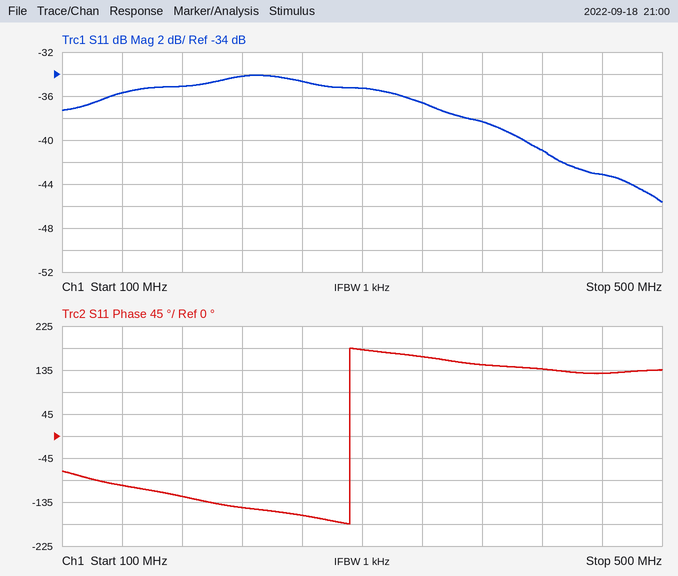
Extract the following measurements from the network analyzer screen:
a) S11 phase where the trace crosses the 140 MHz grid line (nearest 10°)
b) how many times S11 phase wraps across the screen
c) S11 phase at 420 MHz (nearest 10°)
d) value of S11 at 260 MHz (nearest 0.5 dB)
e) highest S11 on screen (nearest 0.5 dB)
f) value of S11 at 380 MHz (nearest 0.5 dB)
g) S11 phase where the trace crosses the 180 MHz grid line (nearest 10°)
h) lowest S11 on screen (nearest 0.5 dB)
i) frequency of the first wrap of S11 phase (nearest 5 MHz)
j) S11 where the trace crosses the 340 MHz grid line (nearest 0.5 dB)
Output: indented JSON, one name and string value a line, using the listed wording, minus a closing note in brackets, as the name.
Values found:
{
  "S11 phase where the trace crosses the 140 MHz grid line": "-100°",
  "how many times S11 phase wraps across the screen": "1",
  "S11 phase at 420 MHz": "140°",
  "value of S11 at 260 MHz": "-34.5 dB",
  "highest S11 on screen": "-34.0 dB",
  "value of S11 at 380 MHz": "-38.5 dB",
  "S11 phase where the trace crosses the 180 MHz grid line": "-120°",
  "lowest S11 on screen": "-45.5 dB",
  "frequency of the first wrap of S11 phase": "290 MHz",
  "S11 where the trace crosses the 340 MHz grid line": "-36.5 dB"
}
